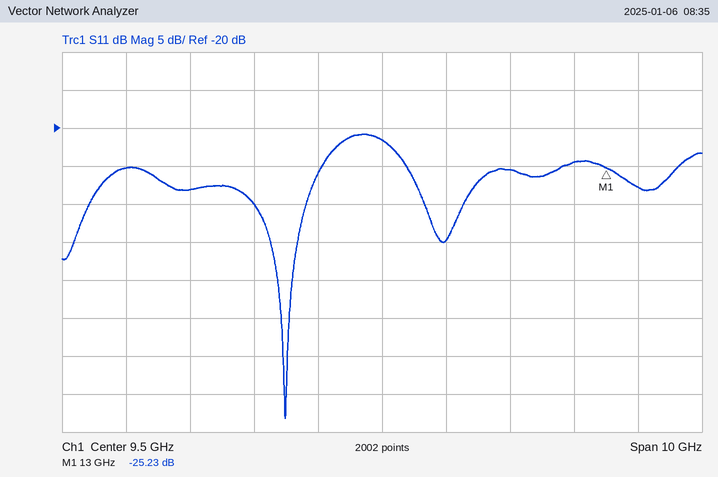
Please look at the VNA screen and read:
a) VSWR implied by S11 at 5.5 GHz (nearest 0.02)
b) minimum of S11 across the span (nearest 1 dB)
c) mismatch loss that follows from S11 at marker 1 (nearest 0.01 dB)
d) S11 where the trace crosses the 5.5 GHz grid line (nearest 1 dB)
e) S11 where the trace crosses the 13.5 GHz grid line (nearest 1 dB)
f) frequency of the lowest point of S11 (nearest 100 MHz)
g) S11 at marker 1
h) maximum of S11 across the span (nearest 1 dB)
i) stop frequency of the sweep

1.12
-58 dB
0.01 dB
-25 dB
-28 dB
8.0 GHz
-25.23 dB
-21 dB
14.5 GHz
